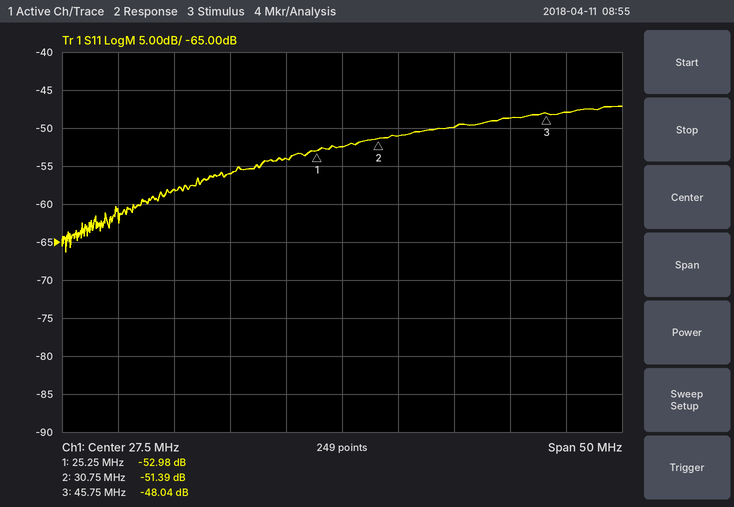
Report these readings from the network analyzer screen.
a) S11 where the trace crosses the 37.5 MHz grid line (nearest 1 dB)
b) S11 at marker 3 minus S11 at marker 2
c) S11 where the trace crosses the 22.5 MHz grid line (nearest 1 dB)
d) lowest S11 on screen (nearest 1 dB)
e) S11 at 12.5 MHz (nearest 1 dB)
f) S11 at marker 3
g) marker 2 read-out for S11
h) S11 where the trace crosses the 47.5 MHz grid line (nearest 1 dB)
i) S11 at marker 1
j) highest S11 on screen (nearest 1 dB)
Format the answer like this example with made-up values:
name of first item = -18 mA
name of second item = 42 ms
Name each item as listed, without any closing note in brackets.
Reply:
S11 where the trace crosses the 37.5 MHz grid line = -50 dB
S11 at marker 3 minus S11 at marker 2 = 3.35 dB
S11 where the trace crosses the 22.5 MHz grid line = -54 dB
lowest S11 on screen = -66 dB
S11 at 12.5 MHz = -58 dB
S11 at marker 3 = -48.04 dB
marker 2 read-out for S11 = -51.39 dB
S11 where the trace crosses the 47.5 MHz grid line = -48 dB
S11 at marker 1 = -52.98 dB
highest S11 on screen = -47 dB
